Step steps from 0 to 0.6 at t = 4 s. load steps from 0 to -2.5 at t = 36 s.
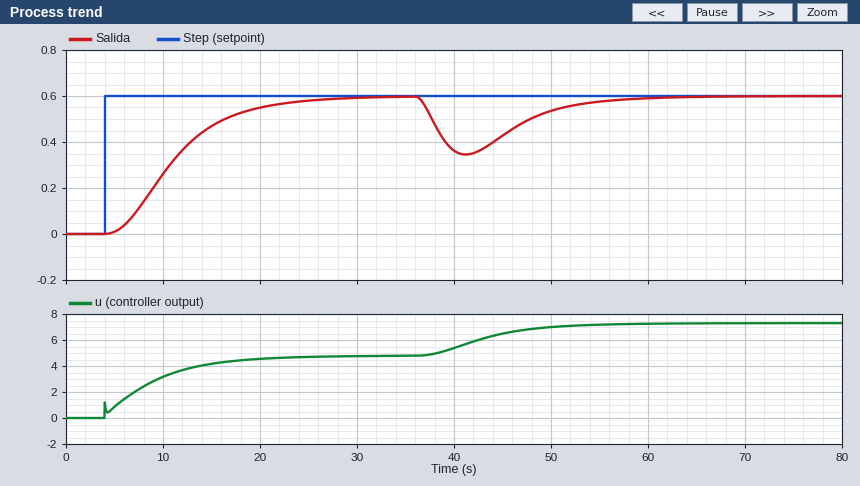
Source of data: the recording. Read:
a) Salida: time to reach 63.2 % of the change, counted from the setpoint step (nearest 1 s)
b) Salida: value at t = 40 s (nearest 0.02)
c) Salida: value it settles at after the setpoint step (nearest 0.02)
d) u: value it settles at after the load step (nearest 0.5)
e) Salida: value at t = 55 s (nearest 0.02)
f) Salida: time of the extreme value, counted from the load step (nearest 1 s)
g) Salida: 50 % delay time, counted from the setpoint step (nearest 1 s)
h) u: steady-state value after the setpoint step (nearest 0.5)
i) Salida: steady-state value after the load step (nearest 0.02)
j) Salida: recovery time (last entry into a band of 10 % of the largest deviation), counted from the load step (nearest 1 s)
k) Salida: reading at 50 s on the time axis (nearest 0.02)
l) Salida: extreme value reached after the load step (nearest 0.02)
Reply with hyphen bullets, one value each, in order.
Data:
- 8 s
- 0.36
- 0.60
- 7.5
- 0.58
- 5 s
- 7 s
- 5.0
- 0.60
- 19 s
- 0.54
- 0.34
